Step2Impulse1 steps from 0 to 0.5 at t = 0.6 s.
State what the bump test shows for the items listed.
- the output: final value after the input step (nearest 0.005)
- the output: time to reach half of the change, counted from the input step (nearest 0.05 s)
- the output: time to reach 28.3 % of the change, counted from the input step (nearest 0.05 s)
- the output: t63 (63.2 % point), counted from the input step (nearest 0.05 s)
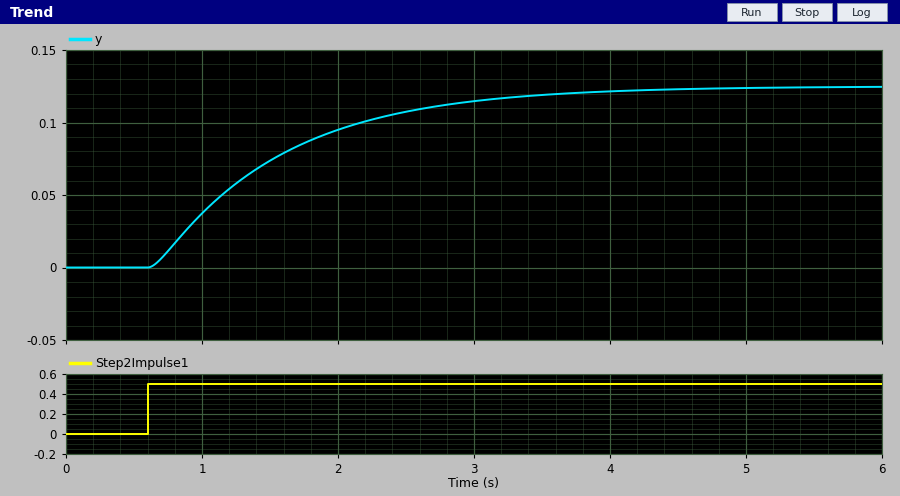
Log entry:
0.125
0.70 s
0.40 s
1.00 s
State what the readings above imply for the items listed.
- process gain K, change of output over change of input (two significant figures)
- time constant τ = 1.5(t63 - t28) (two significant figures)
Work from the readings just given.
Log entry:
0.25
0.90 s
